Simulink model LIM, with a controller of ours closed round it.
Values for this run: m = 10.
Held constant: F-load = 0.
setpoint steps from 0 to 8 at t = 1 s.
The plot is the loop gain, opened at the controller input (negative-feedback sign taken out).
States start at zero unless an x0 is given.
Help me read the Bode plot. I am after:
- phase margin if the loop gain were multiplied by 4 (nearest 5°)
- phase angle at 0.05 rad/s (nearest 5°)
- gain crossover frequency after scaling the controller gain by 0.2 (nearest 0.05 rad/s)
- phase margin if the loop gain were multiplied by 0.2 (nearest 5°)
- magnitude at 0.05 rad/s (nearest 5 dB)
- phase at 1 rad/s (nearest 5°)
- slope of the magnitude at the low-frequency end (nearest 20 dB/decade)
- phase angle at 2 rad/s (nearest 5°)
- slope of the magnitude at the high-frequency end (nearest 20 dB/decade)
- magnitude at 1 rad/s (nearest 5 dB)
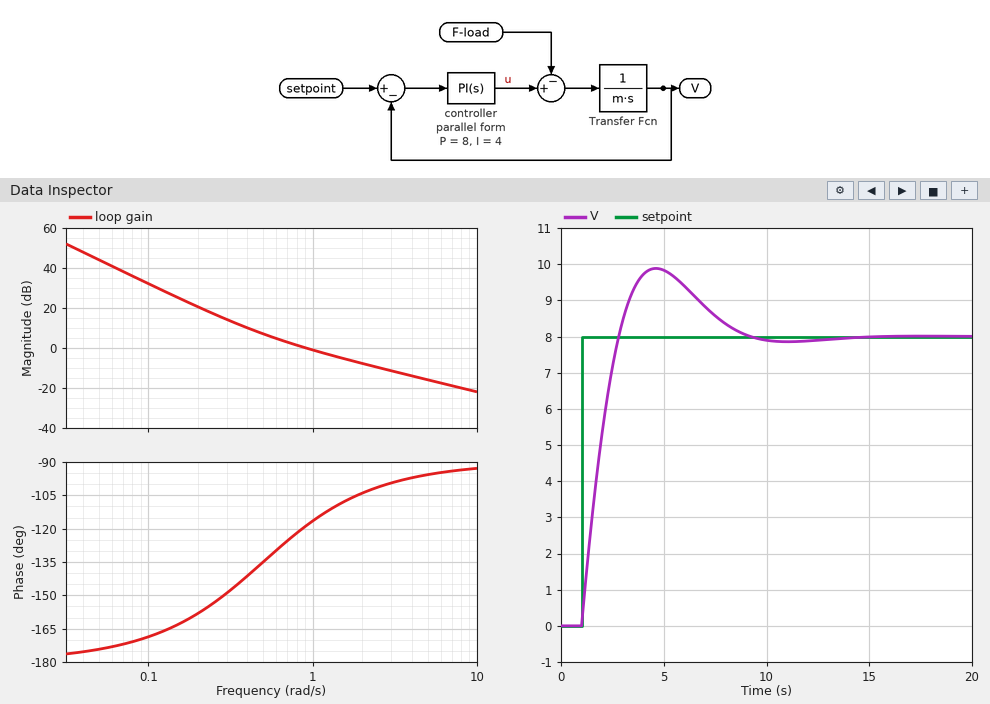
80°
-175°
0.30 rad/s
30°
45 dB
-115°
-40 dB/decade
-105°
-20 dB/decade
0 dB
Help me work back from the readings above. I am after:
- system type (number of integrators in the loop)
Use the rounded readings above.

2
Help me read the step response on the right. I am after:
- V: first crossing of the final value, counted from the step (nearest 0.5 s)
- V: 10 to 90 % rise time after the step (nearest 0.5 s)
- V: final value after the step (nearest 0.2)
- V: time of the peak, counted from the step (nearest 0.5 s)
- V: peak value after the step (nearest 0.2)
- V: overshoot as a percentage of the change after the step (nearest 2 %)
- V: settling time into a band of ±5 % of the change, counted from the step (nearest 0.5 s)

2.0 s
1.5 s
8.0
3.5 s
9.8
24 %
7.0 s
